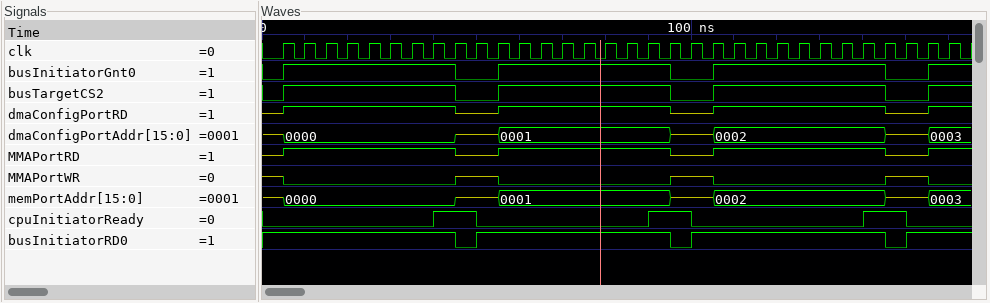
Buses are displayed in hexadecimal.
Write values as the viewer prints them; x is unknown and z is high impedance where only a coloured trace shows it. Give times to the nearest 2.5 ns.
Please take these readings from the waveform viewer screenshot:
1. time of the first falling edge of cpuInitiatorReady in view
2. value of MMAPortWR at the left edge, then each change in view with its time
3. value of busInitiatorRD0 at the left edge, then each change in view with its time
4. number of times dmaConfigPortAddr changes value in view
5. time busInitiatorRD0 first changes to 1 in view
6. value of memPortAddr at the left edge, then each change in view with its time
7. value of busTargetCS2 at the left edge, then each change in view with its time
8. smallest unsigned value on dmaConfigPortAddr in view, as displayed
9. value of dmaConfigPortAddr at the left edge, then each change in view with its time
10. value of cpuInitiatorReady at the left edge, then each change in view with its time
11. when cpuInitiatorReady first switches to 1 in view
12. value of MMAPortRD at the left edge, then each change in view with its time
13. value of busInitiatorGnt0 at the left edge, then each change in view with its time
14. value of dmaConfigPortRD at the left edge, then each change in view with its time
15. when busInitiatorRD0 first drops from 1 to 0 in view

50 ns
z, 0 at 5 ns, z at 45 ns, 0 at 55 ns, z at 95 ns, 0 at 105 ns, z at 145 ns, 0 at 155 ns
1, 0 at 45 ns, 1 at 50 ns, 0 at 95 ns, 1 at 100 ns, 0 at 145 ns, 1 at 150 ns
7
50 ns
z, 0000 at 5 ns, z at 45 ns, 0001 at 55 ns, z at 95 ns, 0002 at 105 ns, z at 145 ns, 0003 at 155 ns
0, 1 at 5 ns, 0 at 45 ns, 1 at 55 ns, 0 at 95 ns, 1 at 105 ns, 0 at 145 ns, 1 at 155 ns
0000
z, 0000 at 5 ns, z at 45 ns, 0001 at 55 ns, z at 95 ns, 0002 at 105 ns, z at 145 ns, 0003 at 155 ns
0, 1 at 40 ns, 0 at 50 ns, 1 at 90 ns, 0 at 100 ns, 1 at 140 ns, 0 at 150 ns
40 ns
z, 1 at 5 ns, z at 45 ns, 1 at 55 ns, z at 95 ns, 1 at 105 ns, z at 145 ns, 1 at 155 ns
0, 1 at 5 ns, 0 at 45 ns, 1 at 55 ns, 0 at 95 ns, 1 at 105 ns, 0 at 145 ns, 1 at 155 ns
z, 1 at 5 ns, z at 45 ns, 1 at 55 ns, z at 95 ns, 1 at 105 ns, z at 145 ns, 1 at 155 ns
45 ns
